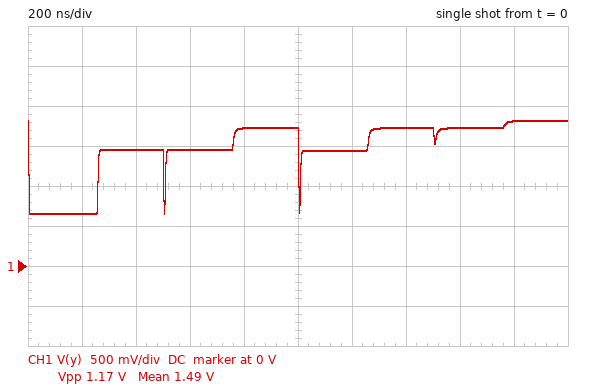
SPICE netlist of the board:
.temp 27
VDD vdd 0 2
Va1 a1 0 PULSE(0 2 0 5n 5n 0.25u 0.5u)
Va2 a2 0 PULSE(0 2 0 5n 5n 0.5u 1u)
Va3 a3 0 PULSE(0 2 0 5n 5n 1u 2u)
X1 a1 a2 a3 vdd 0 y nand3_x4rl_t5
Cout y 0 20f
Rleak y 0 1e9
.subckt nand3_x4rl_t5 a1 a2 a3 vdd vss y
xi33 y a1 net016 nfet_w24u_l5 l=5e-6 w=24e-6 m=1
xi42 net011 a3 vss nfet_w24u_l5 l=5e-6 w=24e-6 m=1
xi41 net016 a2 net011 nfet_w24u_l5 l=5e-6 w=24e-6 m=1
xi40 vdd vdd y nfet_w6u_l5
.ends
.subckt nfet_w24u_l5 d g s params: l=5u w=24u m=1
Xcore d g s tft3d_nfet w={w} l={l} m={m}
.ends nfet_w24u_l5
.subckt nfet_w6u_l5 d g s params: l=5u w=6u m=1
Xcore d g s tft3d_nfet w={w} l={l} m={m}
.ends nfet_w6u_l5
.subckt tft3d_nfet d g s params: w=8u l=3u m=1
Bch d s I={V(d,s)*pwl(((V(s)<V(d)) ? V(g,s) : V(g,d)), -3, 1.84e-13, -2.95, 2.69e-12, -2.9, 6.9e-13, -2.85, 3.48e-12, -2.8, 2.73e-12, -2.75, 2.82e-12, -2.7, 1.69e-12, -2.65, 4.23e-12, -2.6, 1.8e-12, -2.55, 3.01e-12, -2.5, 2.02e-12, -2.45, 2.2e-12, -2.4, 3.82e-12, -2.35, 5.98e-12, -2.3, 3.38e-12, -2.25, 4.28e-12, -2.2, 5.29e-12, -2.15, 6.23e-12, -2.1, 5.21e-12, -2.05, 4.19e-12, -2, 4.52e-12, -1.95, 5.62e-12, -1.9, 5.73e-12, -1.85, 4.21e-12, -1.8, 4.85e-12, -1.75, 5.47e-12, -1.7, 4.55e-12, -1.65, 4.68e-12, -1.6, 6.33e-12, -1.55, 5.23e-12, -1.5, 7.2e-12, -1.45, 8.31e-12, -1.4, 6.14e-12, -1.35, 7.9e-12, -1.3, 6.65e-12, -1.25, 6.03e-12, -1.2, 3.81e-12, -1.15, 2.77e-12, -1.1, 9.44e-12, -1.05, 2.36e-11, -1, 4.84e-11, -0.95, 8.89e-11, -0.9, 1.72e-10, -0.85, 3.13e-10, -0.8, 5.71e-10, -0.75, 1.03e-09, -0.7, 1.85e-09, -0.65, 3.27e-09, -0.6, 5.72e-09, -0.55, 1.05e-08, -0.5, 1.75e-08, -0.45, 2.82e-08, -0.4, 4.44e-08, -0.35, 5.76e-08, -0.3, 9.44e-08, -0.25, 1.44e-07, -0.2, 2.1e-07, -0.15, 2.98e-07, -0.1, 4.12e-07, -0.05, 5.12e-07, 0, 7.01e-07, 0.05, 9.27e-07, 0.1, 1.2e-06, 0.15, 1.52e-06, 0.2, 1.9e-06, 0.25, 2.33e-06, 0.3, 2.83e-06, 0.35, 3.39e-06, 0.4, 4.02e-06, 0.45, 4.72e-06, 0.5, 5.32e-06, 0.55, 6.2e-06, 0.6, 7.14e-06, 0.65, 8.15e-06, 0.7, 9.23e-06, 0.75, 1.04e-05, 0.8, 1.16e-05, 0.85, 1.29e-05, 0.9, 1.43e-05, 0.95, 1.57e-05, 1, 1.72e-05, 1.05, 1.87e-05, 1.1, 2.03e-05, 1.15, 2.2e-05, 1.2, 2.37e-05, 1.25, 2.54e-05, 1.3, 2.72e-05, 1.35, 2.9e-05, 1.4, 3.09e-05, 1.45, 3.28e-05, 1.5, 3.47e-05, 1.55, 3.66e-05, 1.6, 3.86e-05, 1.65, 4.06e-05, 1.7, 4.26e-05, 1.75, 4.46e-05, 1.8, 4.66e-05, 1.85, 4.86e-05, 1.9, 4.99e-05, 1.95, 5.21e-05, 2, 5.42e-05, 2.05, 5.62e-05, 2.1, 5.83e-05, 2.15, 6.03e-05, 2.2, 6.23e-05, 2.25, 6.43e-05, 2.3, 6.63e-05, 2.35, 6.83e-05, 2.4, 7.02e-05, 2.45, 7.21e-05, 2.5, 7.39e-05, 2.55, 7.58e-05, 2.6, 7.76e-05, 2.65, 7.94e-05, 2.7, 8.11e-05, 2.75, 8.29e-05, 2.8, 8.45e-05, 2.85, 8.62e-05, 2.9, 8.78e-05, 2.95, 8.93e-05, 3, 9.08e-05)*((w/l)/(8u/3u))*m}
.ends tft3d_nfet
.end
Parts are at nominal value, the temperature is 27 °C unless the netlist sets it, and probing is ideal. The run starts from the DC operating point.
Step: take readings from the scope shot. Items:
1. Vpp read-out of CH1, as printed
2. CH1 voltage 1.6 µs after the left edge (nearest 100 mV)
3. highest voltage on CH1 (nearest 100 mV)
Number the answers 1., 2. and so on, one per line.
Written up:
1. 1.17 V
2. 1.7 V
3. 1.8 V
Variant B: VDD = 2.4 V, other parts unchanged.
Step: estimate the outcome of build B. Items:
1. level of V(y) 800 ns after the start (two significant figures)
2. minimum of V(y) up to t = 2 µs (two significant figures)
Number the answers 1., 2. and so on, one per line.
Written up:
1. 2.1 V
2. 900 mV
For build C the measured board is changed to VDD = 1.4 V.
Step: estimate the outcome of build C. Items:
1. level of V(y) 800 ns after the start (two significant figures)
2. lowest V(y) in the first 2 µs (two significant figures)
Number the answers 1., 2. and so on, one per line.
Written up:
1. 1.1 V
2. 320 mV
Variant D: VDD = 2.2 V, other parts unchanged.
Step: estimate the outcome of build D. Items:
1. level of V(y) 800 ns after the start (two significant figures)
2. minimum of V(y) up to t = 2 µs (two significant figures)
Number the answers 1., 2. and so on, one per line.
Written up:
1. 1.9 V
2. 770 mV
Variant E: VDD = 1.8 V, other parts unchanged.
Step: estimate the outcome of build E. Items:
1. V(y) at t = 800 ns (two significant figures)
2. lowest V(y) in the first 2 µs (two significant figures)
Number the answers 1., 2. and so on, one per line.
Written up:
1. 1.5 V
2. 530 mV
